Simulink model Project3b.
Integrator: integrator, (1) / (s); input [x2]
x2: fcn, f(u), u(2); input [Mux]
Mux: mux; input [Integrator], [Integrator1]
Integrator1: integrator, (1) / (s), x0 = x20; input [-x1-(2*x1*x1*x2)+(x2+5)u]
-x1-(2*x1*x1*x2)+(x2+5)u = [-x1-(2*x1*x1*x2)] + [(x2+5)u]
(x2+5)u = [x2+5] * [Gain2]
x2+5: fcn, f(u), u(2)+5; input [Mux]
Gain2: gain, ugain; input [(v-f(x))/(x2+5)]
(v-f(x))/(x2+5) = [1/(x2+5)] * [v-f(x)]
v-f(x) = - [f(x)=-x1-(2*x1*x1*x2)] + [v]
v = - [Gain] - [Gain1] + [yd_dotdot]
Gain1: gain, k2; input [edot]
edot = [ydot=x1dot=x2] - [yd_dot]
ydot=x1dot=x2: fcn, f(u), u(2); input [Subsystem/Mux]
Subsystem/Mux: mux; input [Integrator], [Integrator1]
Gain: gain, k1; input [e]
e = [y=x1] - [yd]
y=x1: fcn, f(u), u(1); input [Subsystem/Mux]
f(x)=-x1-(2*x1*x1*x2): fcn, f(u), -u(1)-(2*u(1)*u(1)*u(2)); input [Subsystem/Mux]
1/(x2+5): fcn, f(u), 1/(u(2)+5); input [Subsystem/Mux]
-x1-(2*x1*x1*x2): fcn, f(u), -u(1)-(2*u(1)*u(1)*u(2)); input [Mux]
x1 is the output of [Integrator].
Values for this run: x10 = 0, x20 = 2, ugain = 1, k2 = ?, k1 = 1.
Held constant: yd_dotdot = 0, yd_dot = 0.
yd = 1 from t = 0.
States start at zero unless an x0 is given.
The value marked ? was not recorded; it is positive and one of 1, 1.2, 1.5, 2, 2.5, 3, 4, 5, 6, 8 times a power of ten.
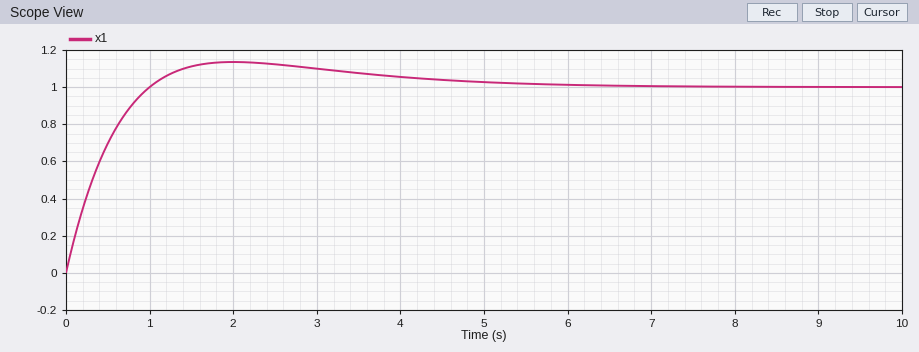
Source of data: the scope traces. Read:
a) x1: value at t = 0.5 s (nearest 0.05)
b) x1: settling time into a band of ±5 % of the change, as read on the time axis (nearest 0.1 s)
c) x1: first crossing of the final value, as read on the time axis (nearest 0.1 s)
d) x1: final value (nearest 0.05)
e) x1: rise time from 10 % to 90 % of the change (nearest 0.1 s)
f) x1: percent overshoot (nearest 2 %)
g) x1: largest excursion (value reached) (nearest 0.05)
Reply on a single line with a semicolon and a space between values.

0.70; 4.1 s; 1.0 s; 1.00; 0.7 s; 14 %; 1.15
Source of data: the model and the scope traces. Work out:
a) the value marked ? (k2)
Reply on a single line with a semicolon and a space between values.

2
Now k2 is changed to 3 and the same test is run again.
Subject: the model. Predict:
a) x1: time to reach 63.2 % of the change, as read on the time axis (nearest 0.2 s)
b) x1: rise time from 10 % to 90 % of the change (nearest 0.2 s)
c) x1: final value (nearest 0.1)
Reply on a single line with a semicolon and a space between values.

0.6 s; 2.6 s; 1.0
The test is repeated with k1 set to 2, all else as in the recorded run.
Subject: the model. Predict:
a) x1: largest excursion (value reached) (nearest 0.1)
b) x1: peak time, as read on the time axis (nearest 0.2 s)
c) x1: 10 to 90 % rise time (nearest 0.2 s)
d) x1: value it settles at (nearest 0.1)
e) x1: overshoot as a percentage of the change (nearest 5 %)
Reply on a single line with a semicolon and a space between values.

1.2; 1.6 s; 0.6 s; 1.0; 20 %
